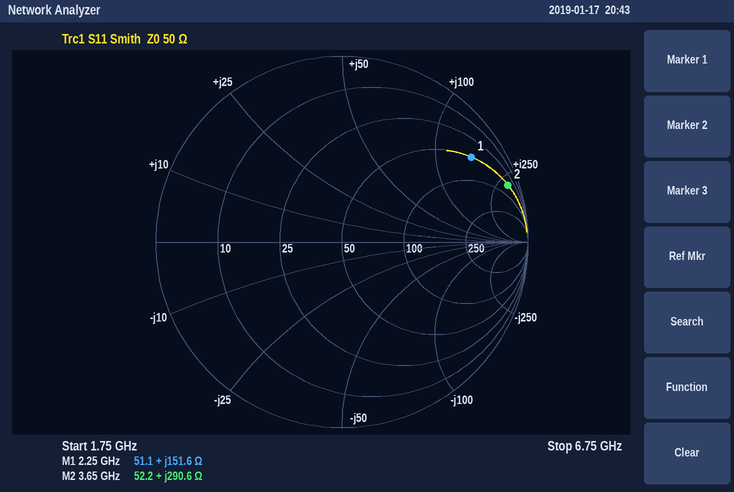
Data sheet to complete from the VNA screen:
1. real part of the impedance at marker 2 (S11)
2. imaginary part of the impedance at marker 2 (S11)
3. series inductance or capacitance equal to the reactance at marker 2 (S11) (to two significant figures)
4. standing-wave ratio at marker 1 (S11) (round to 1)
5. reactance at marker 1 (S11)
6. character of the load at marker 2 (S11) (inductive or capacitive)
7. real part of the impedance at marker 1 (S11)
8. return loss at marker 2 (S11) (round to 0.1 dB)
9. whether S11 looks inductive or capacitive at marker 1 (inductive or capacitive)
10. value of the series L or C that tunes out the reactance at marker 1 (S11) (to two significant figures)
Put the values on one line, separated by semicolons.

52.2 Ω; +290.6 Ω; 13 nH; 11; +151.6 Ω; inductive; 51.1 Ω; 0.5 dB; inductive; 470 fF
